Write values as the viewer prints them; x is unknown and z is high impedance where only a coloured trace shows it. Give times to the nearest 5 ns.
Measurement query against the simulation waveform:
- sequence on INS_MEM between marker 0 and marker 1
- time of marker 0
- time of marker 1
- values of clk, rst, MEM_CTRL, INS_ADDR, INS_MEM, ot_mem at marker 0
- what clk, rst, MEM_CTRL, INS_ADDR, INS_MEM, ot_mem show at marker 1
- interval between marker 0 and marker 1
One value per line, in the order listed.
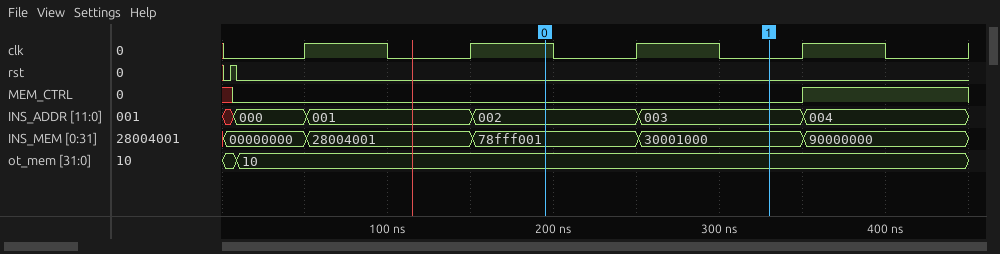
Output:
78fff001, 30001000
195 ns
330 ns
clk=1, rst=0, MEM_CTRL=0, INS_ADDR=002, INS_MEM=78fff001, ot_mem=10
clk=0, rst=0, MEM_CTRL=0, INS_ADDR=003, INS_MEM=30001000, ot_mem=10
135 ns
